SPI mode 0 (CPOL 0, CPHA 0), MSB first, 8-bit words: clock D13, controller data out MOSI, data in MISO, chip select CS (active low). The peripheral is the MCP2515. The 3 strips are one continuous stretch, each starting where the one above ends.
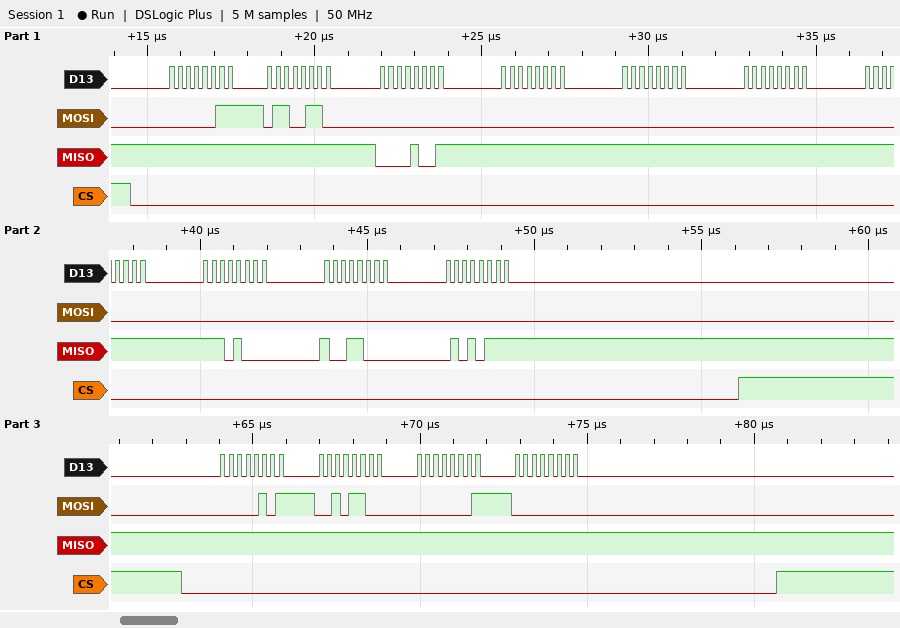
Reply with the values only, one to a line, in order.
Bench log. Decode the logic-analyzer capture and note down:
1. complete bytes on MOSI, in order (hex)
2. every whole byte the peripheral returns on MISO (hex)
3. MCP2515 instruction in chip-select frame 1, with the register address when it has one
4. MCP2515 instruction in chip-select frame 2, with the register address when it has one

03 66 00 00 00 00 00 00 00 00 05 2C 01 00
FF FF 09 FF FF FF FF E8 98 57 FF FF FF FF
READ 0x66
BIT MODIFY 0x2C
